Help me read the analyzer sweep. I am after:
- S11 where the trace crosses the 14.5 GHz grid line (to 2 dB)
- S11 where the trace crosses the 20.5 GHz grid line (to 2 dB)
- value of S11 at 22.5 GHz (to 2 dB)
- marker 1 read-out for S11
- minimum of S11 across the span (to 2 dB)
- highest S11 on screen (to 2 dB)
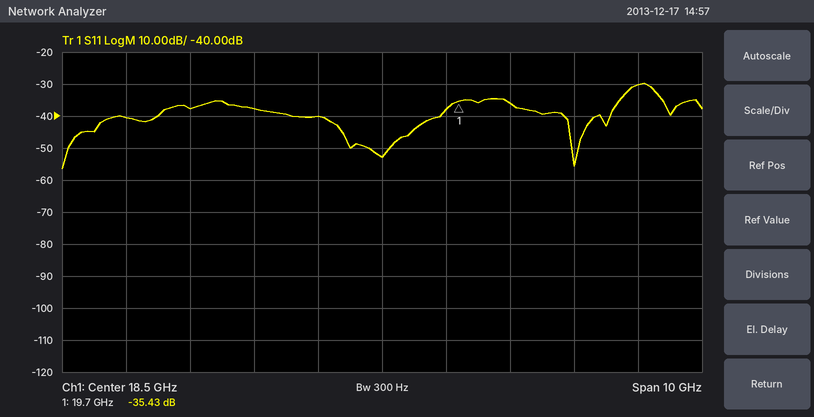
-40 dB
-36 dB
-30 dB
-35.43 dB
-56 dB
-30 dB
